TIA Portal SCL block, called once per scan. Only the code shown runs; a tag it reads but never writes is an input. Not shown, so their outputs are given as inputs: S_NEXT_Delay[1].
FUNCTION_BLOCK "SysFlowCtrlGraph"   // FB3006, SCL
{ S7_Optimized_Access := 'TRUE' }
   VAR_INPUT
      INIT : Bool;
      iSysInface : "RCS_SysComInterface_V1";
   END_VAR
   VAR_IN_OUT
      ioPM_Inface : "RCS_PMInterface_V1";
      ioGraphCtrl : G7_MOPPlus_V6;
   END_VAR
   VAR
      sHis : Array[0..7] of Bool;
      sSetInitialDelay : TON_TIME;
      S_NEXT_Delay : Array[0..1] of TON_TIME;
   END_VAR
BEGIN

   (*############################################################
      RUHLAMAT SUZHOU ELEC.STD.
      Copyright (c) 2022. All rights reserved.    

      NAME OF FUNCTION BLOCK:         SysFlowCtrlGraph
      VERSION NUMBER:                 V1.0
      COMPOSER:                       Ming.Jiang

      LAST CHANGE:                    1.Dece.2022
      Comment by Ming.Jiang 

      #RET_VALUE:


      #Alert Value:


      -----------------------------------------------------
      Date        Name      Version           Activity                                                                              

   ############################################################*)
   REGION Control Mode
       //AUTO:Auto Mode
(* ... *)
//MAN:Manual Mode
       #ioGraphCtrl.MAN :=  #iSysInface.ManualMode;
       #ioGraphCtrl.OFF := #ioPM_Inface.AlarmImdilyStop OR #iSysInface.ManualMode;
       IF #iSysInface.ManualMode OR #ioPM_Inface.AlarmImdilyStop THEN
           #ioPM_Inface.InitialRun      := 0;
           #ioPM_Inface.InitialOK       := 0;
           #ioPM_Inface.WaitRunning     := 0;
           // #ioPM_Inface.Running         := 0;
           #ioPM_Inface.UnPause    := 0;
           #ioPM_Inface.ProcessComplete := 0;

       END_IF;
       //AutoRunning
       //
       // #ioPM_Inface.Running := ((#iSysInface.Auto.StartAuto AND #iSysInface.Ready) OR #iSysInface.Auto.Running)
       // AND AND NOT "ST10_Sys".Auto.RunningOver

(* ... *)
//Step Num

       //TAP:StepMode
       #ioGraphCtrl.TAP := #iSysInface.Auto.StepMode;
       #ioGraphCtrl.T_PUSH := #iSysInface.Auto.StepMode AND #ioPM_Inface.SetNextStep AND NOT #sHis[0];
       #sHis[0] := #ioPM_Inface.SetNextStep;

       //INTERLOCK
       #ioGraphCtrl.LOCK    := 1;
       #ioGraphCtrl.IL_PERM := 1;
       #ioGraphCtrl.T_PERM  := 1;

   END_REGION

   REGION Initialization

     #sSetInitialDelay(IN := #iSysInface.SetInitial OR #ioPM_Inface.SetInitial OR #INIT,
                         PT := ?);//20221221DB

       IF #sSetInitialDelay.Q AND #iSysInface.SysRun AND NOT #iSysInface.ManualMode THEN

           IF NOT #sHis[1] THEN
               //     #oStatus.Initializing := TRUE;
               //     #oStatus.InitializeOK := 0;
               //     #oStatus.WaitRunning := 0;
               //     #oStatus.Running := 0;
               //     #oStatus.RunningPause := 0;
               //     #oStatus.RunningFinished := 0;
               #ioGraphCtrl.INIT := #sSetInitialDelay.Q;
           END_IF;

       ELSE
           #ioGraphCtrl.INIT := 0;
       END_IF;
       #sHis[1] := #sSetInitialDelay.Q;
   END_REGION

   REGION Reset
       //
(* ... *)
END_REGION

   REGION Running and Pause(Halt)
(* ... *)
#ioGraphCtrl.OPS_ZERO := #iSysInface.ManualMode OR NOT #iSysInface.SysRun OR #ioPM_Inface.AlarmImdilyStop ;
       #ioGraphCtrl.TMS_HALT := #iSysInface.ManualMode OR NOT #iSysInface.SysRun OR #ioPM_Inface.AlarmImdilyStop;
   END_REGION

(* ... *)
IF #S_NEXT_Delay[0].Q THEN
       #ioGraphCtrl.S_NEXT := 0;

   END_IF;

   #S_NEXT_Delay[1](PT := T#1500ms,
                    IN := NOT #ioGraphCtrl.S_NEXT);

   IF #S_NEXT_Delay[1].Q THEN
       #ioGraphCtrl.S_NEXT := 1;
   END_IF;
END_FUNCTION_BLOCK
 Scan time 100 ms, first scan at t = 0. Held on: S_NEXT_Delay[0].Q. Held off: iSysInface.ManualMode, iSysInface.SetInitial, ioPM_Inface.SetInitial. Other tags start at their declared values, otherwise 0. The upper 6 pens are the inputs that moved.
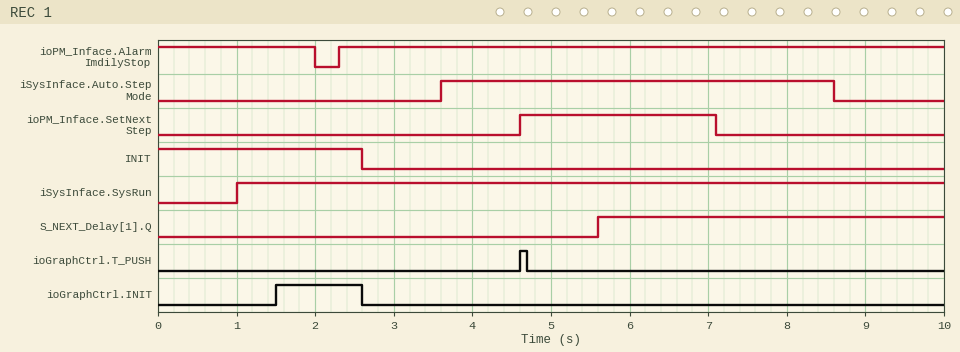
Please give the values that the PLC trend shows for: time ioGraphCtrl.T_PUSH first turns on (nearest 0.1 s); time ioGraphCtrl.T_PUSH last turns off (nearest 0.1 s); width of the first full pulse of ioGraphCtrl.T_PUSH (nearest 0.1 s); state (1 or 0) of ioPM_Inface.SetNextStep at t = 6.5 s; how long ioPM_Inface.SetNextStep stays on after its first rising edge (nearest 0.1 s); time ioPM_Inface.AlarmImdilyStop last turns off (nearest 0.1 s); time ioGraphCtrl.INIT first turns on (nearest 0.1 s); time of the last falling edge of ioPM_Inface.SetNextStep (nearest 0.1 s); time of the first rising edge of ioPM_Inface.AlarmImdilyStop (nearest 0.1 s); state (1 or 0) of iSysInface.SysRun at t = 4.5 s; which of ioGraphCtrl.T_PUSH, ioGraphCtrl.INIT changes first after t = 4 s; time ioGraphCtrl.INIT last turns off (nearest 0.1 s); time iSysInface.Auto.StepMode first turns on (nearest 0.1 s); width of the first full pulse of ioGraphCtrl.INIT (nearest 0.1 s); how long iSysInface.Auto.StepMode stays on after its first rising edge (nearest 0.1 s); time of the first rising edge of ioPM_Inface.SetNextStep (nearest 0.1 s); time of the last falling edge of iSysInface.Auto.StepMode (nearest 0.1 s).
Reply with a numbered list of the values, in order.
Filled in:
1. 4.6 s
2. 4.7 s
3. 0.1 s
4. 1
5. 2.5 s
6. 2.0 s
7. 1.5 s
8. 7.1 s
9. 2.3 s
10. 1
11. ioGraphCtrl.T_PUSH
12. 2.6 s
13. 3.6 s
14. 1.1 s
15. 5.0 s
16. 4.6 s
17. 8.6 s
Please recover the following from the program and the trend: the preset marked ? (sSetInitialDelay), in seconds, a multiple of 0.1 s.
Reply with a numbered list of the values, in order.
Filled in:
1. 1.5 s
